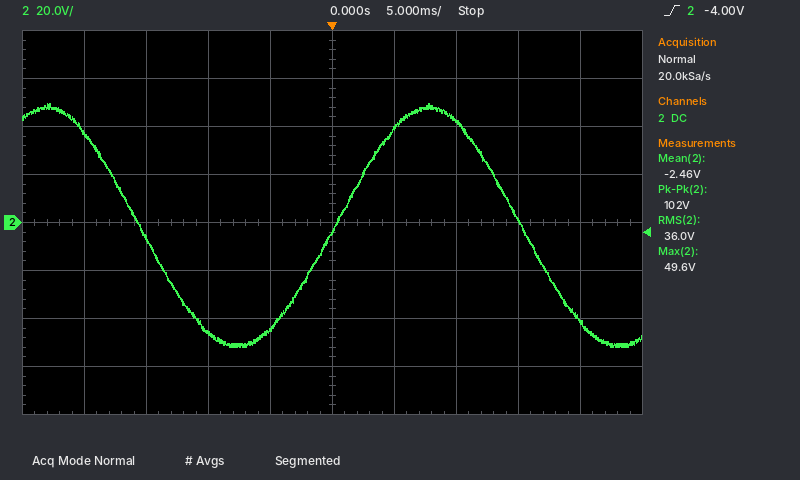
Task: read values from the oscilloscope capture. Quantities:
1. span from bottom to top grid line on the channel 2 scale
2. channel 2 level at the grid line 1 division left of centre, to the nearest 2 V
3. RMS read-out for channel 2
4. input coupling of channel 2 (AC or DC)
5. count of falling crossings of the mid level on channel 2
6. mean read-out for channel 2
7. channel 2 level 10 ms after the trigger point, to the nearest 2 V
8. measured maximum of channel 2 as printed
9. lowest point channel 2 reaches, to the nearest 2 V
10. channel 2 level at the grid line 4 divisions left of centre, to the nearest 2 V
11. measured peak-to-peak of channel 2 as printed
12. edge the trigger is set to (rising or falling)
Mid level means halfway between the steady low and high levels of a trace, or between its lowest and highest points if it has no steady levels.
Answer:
160 V
-44 V
36.0 V
DC
2
-2.46 V
42 V
49.6 V
-52 V
38 V
102 V
rising
